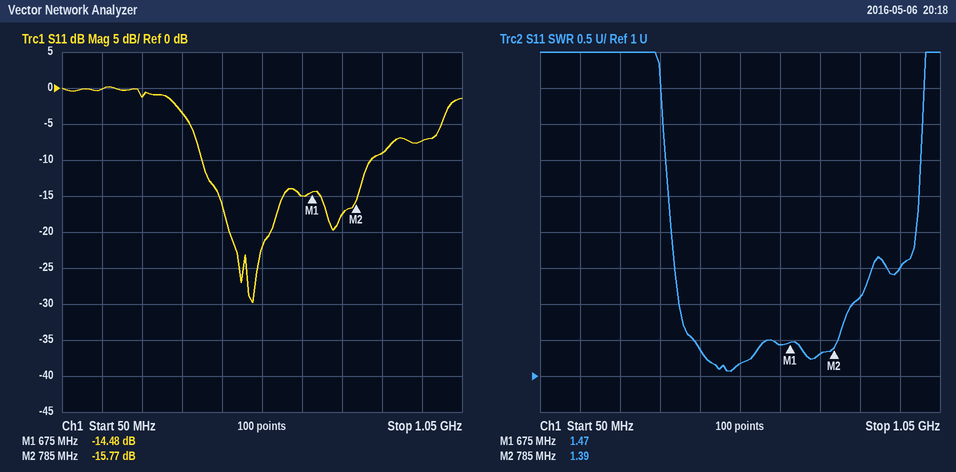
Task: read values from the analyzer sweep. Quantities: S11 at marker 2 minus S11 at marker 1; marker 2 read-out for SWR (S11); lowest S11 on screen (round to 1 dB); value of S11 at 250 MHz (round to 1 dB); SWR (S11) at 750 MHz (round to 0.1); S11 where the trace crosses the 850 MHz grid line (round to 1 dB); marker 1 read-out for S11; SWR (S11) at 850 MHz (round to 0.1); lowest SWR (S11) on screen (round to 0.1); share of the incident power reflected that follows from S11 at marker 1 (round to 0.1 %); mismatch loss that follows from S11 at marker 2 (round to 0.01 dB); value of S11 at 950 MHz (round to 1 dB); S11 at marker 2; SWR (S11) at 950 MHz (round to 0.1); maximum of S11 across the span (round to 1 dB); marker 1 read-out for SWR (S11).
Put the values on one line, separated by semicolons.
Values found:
-1.29 dB; 1.39; -30 dB; -1 dB; 1.3; -9 dB; -14.48 dB; 2.1; 1.1; 3.6 %; 0.12 dB; -7 dB; -15.77 dB; 2.5; 0 dB; 1.47
